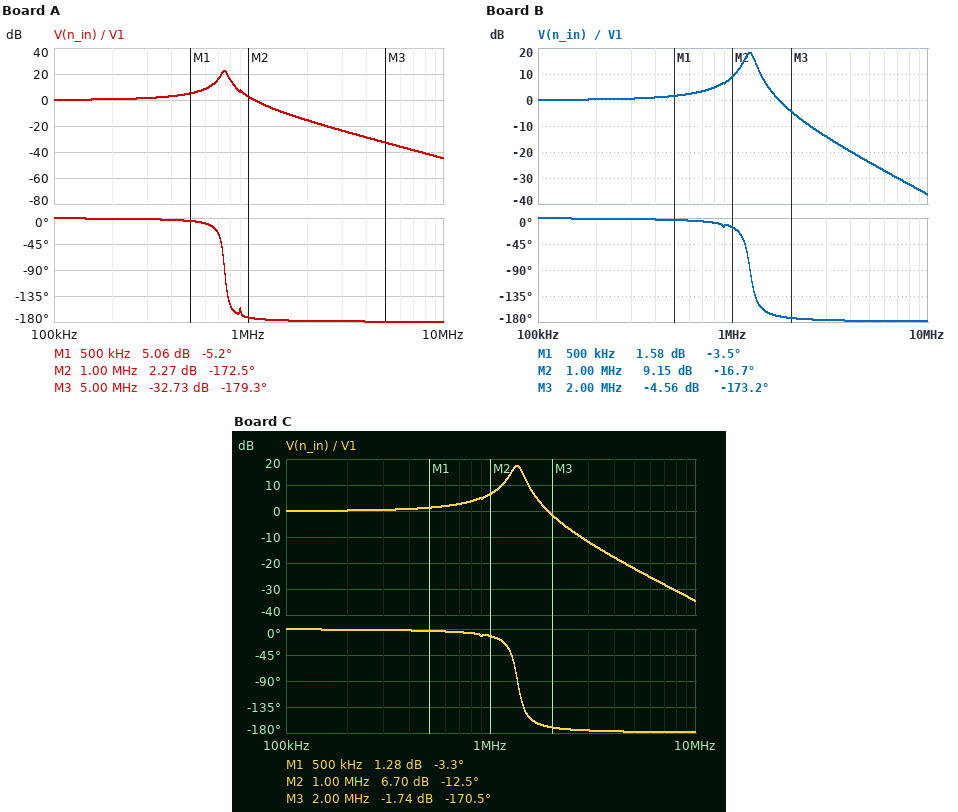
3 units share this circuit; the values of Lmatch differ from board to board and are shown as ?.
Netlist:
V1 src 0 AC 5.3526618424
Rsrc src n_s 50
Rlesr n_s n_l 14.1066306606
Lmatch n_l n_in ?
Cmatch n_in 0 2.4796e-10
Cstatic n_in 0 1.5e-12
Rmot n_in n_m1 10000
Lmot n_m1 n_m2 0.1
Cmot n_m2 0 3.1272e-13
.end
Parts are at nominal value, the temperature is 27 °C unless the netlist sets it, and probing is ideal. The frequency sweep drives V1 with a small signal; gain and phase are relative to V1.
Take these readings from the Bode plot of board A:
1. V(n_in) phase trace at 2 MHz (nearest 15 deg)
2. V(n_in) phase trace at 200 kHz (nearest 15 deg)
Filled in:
-180 deg
0 deg
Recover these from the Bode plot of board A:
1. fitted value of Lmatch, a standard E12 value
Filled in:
180 µH
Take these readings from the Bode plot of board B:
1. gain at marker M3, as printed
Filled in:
-4.56 dB
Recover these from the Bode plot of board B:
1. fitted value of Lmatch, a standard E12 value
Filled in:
68 µH
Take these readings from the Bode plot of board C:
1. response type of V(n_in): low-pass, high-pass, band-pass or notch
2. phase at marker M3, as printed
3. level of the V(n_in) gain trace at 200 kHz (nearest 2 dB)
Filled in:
low-pass
-170.5 deg
0 dB
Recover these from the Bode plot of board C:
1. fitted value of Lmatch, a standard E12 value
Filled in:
56 µH
